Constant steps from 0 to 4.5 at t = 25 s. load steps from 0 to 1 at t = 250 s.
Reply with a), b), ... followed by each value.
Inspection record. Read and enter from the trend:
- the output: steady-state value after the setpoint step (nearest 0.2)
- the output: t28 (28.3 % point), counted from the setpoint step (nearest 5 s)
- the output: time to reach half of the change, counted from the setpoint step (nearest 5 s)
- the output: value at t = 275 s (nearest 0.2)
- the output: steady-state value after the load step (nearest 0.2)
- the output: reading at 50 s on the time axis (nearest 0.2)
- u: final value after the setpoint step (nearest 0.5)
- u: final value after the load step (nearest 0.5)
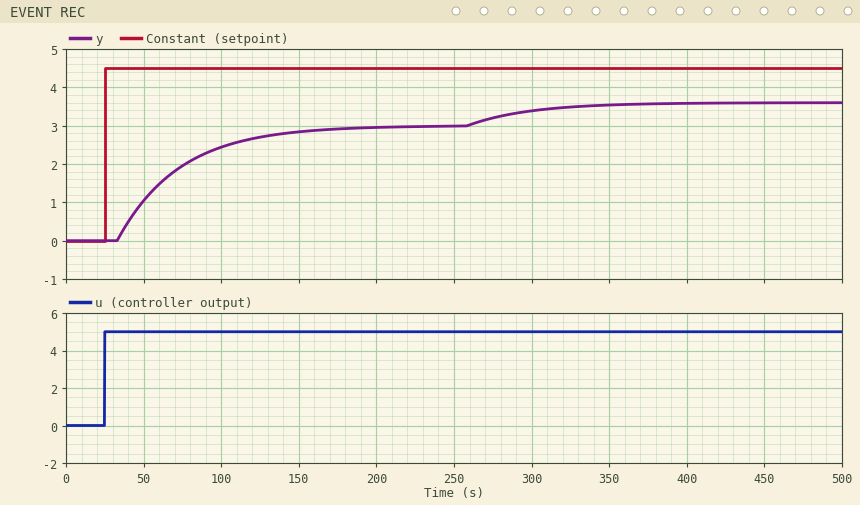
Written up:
a) 3.0
b) 20 s
c) 35 s
d) 3.2
e) 3.6
f) 1.0
g) 5.0
h) 5.0
